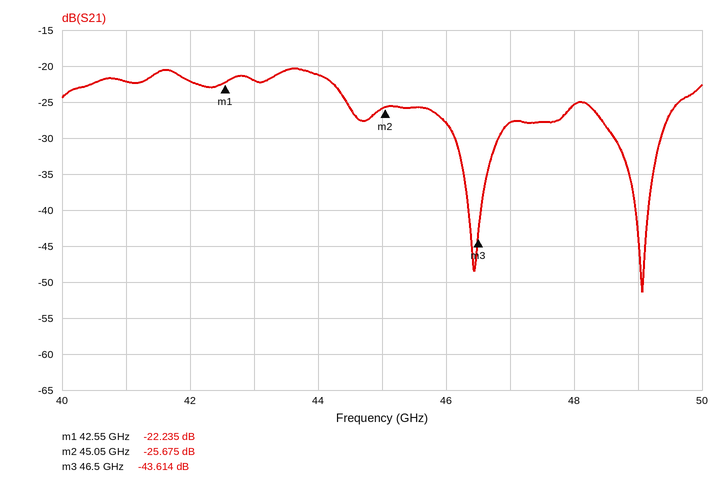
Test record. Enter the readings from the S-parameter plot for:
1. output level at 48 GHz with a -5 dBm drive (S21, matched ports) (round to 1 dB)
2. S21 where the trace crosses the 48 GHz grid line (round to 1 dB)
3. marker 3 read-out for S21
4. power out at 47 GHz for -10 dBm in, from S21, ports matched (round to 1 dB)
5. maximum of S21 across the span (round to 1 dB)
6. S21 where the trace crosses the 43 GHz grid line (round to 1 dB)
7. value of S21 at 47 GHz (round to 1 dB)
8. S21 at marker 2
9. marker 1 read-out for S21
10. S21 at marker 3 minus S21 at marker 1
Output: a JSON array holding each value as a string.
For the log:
["-30 dBm", "-25 dB", "-43.614 dB", "-38 dBm", "-20 dB", "-22 dB", "-28 dB", "-25.675 dB", "-22.235 dB", "-21.379 dB"]
